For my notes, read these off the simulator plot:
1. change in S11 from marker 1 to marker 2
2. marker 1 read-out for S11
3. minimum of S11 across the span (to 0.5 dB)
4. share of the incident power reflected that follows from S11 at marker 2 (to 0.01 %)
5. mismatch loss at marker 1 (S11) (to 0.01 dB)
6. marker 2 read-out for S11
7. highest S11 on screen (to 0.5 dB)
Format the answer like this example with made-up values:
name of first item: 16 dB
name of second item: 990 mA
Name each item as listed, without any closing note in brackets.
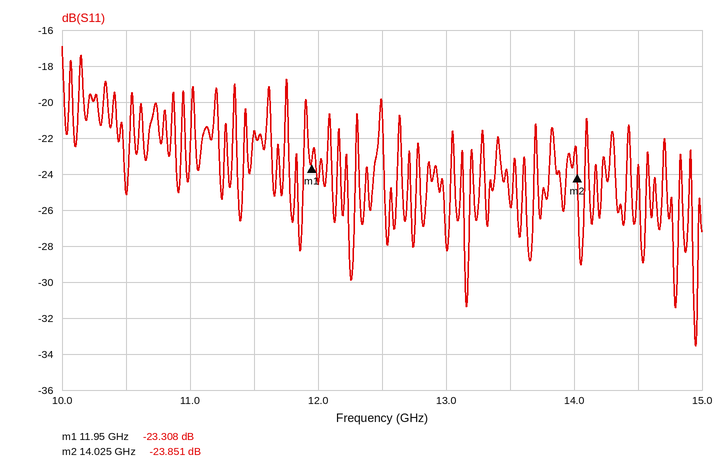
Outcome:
change in S11 from marker 1 to marker 2: -0.543 dB
marker 1 read-out for S11: -23.308 dB
minimum of S11 across the span: -33.5 dB
share of the incident power reflected that follows from S11 at marker 2: 0.41 %
mismatch loss at marker 1 (S11): 0.02 dB
marker 2 read-out for S11: -23.851 dB
highest S11 on screen: -17.0 dB
